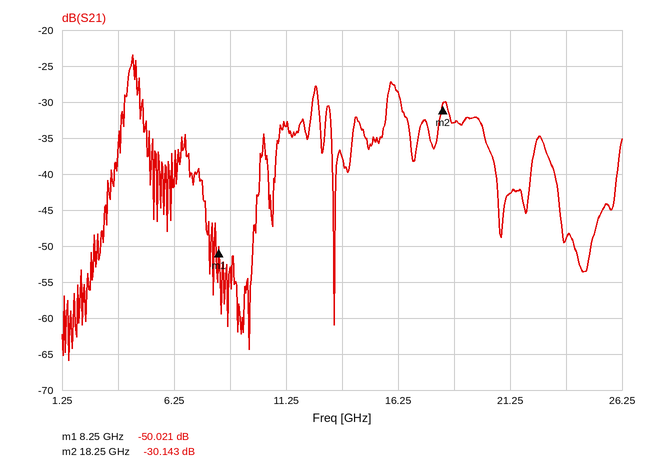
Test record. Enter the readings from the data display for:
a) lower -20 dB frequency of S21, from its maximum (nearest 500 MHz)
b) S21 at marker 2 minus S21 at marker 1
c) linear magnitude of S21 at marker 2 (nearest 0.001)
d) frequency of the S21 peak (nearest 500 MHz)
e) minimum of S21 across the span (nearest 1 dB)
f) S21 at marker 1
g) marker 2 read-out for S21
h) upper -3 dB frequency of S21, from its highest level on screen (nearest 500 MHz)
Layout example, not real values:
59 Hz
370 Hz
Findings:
3.5 GHz
19.878 dB
0.031
4.5 GHz
-66 dB
-50.021 dB
-30.143 dB
4.5 GHz
